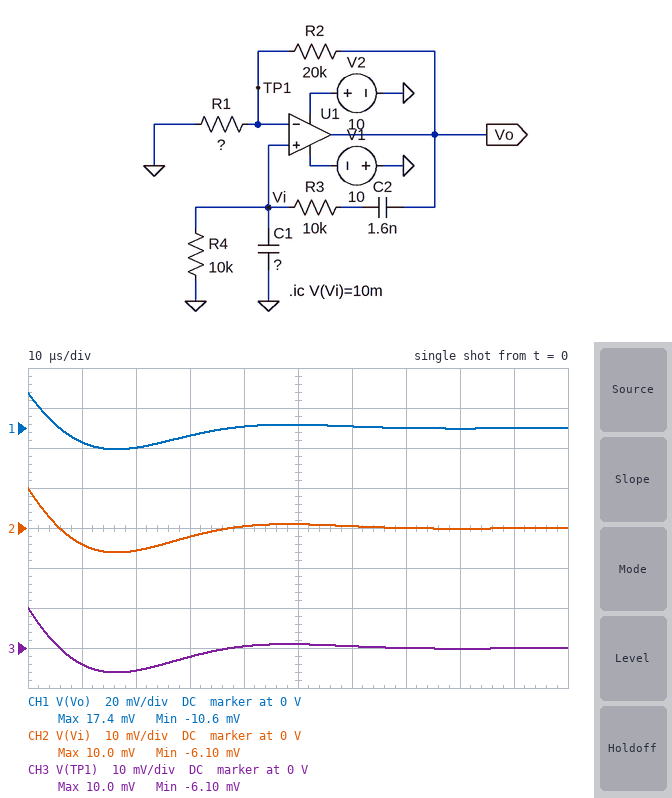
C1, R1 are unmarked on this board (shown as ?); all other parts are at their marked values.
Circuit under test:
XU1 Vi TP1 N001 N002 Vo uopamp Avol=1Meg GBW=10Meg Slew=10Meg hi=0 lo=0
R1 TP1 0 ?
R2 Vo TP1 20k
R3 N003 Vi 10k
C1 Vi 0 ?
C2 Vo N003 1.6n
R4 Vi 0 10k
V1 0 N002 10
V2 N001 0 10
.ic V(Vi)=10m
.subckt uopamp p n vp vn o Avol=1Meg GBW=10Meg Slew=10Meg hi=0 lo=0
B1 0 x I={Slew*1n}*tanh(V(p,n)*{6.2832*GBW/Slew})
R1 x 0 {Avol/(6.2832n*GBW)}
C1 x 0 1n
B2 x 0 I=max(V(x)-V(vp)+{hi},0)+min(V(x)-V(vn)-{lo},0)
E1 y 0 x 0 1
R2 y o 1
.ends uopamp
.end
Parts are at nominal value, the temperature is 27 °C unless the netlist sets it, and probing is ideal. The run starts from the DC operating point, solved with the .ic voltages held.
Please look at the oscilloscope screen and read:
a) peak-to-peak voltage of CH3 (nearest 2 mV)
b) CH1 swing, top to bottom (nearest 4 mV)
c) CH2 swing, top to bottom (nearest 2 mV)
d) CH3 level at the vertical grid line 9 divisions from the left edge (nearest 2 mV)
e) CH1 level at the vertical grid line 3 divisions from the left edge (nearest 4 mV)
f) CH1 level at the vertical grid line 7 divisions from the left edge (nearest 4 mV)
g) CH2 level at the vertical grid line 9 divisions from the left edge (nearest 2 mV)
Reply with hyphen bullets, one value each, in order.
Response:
- 16 mV
- 28 mV
- 16 mV
- 0 V
- -4 mV
- 0 V
- 0 V
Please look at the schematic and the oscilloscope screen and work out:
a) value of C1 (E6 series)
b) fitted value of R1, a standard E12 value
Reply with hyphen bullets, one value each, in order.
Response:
- 470 pF
- 27 kΩ
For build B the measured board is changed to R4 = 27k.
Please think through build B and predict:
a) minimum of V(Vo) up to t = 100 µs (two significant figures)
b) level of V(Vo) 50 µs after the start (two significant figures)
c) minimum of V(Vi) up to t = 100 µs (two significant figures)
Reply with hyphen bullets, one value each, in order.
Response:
- -36 mV
- -14 mV
- -21 mV
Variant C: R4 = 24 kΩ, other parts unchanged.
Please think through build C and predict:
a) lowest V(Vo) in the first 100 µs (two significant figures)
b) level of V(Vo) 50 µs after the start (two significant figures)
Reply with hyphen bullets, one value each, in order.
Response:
- -30 mV
- -4.1 mV
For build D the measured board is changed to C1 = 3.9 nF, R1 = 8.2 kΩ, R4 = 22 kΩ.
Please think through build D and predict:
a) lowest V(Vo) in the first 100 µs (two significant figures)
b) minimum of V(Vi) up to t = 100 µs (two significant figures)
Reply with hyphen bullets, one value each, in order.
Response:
- -19 mV
- -5.5 mV
